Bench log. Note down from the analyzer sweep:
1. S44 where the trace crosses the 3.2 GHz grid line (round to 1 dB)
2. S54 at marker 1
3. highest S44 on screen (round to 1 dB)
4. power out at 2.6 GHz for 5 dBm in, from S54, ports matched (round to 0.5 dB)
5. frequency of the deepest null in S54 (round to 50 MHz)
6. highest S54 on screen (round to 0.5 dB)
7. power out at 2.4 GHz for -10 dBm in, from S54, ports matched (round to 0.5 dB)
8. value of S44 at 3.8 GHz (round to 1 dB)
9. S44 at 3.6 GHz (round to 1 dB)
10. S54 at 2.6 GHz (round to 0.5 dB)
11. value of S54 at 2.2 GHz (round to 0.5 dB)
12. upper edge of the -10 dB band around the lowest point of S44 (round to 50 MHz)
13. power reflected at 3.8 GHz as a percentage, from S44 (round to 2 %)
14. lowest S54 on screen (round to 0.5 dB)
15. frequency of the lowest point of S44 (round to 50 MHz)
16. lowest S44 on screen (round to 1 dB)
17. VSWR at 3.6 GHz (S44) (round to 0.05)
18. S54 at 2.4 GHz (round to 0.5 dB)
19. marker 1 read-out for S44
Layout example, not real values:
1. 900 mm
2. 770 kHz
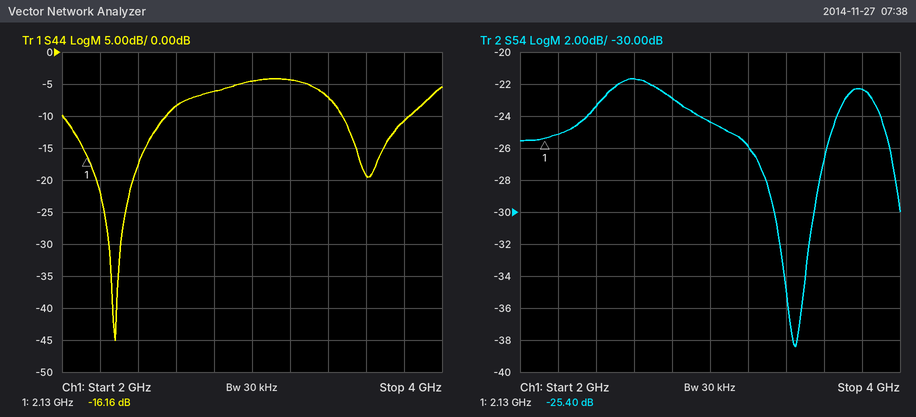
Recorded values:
1. -4 dB
2. -25.40 dB
3. -4 dB
4. -16.5 dBm
5. 3.45 GHz
6. -21.5 dB
7. -33.5 dBm
8. -11 dB
9. -19 dB
10. -21.5 dB
11. -25.0 dB
12. 2.55 GHz
13. 8 %
14. -38.5 dB
15. 2.30 GHz
16. -45 dB
17. 1.25
18. -23.5 dB
19. -16.16 dB
